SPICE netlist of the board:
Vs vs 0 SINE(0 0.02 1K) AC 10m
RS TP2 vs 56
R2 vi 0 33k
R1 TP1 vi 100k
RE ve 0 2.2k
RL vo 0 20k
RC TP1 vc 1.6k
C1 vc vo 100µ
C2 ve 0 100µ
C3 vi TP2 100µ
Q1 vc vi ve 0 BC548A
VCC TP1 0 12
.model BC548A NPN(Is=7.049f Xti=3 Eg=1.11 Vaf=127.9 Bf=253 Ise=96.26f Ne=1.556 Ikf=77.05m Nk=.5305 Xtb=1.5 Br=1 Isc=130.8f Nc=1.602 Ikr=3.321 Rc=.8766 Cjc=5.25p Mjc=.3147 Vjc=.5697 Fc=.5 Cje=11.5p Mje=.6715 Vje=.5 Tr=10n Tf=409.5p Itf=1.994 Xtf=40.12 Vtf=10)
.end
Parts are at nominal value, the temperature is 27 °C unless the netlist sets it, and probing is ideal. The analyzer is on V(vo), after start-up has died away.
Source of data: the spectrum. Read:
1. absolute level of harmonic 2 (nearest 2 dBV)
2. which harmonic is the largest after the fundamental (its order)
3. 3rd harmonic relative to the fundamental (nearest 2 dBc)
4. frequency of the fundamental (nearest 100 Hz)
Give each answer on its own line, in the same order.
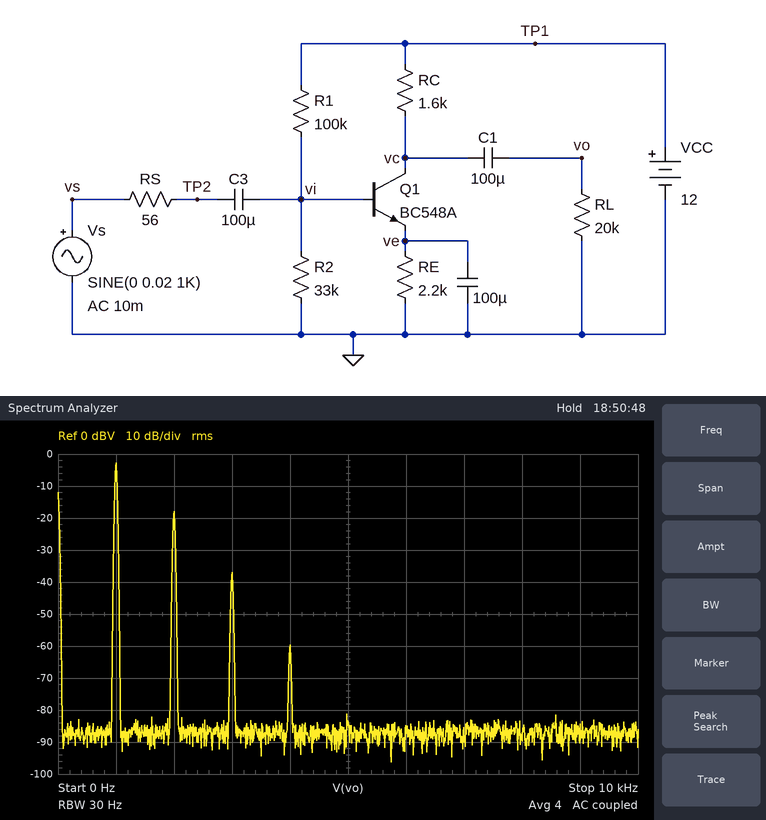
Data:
-18 dBV
2
-34 dBc
1.0 kHz
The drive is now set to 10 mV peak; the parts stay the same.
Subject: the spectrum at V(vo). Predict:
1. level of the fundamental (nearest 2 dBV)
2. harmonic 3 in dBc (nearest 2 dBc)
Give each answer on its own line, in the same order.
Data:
-8 dBV
-46 dBc
